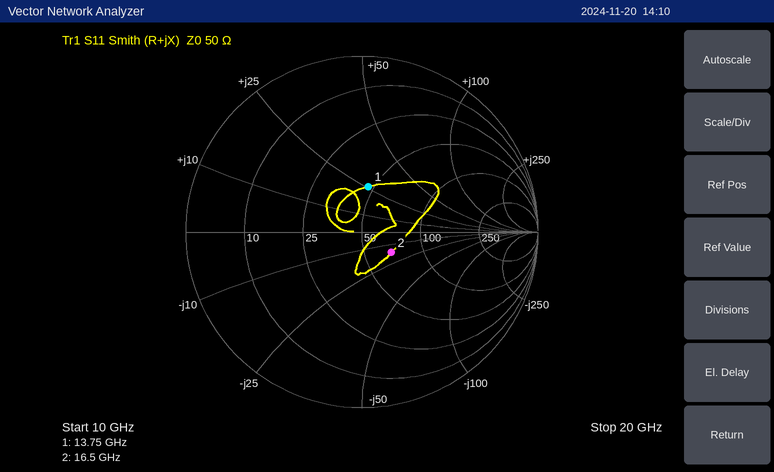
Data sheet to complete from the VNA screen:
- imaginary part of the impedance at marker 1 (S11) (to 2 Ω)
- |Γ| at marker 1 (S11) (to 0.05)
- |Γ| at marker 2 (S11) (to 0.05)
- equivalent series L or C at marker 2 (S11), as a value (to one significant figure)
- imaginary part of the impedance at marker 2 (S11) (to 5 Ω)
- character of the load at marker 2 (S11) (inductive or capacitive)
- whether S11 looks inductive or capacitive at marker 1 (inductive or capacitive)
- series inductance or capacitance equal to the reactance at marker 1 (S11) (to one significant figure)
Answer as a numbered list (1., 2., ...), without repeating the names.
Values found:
1. +26 Ω
2. 0.25
3. 0.20
4. 600 fF
5. -15 Ω
6. capacitive
7. inductive
8. 300 pH
